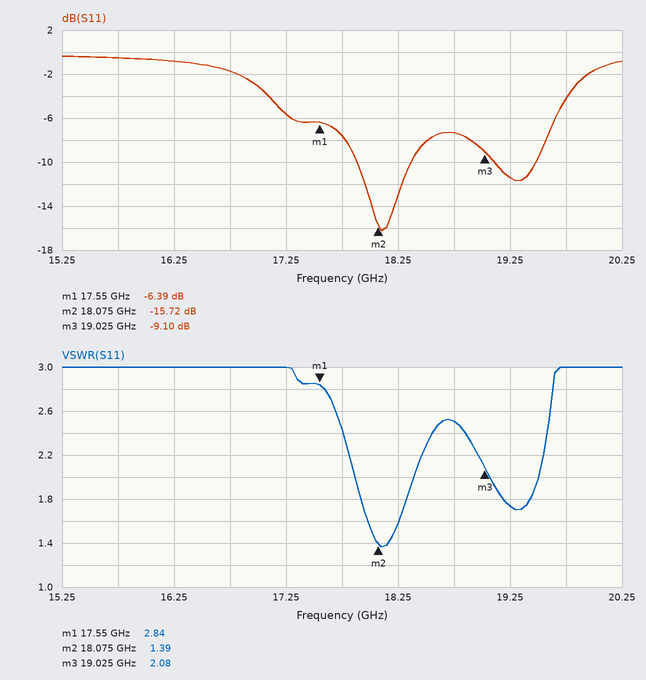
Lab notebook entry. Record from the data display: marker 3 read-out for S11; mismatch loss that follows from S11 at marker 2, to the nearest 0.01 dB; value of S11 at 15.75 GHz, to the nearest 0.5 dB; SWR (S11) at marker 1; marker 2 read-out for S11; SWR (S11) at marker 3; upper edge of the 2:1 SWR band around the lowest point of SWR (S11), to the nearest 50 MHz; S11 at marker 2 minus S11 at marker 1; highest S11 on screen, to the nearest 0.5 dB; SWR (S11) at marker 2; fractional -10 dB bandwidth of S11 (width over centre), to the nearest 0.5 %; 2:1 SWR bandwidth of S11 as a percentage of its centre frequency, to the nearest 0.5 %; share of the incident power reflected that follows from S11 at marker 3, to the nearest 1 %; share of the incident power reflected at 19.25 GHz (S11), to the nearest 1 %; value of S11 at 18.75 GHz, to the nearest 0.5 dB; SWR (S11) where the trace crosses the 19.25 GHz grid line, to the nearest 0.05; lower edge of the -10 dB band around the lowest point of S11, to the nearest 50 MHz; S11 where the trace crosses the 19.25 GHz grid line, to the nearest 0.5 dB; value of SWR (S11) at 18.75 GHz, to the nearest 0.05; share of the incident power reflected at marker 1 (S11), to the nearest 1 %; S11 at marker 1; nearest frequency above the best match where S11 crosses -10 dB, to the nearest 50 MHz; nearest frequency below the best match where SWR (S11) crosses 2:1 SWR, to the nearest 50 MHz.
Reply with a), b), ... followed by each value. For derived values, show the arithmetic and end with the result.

a) -9.10 dB
b) −10 log10(1 − 10^(-15.72/10)) ≈ 0.12 dB
c) -0.5 dB
d) 2.84
e) -15.72 dB
f) 2.08
g) 18.40 GHz
h) -15.72 − (-6.39) = -9.33 dB
i) -0.5 dB
j) 1.39
k) 450 MHz / 18.125 GHz ≈ 2.5 %
l) 550 MHz / 18.125 GHz ≈ 3.0 %
m) 10^(-9.1/10) ≈ 12 %
n) 10^(-11.5/10) ≈ 7 %
o) -7.5 dB
p) 1.75
q) 17.90 GHz
r) -11.5 dB
s) 2.50
t) 10^(-6.39/10) ≈ 23 %
u) -6.39 dB
v) 18.35 GHz
w) 17.85 GHz
